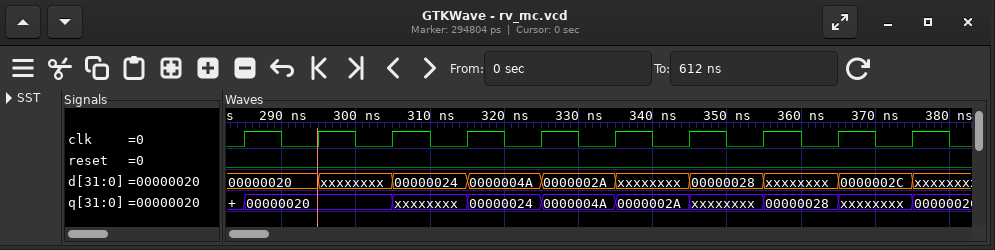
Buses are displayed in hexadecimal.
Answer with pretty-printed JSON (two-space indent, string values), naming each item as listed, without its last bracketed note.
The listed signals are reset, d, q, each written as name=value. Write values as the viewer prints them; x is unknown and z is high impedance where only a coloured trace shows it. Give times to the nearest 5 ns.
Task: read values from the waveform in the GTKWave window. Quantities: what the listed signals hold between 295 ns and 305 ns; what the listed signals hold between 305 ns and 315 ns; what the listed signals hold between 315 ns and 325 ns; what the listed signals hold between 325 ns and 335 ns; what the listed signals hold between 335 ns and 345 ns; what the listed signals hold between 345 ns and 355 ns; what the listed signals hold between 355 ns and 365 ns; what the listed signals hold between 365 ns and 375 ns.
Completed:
{
  "what the listed signals hold between 295 ns and 305 ns": "reset=0, d=xxxxxxxx, q=00000020",
  "what the listed signals hold between 305 ns and 315 ns": "reset=0, d=00000024, q=xxxxxxxx",
  "what the listed signals hold between 315 ns and 325 ns": "reset=0, d=0000004A, q=00000024",
  "what the listed signals hold between 325 ns and 335 ns": "reset=0, d=0000002A, q=0000004A",
  "what the listed signals hold between 335 ns and 345 ns": "reset=0, d=xxxxxxxx, q=0000002A",
  "what the listed signals hold between 345 ns and 355 ns": "reset=0, d=00000028, q=xxxxxxxx",
  "what the listed signals hold between 355 ns and 365 ns": "reset=0, d=xxxxxxxx, q=00000028",
  "what the listed signals hold between 365 ns and 375 ns": "reset=0, d=0000002C, q=xxxxxxxx"
}
